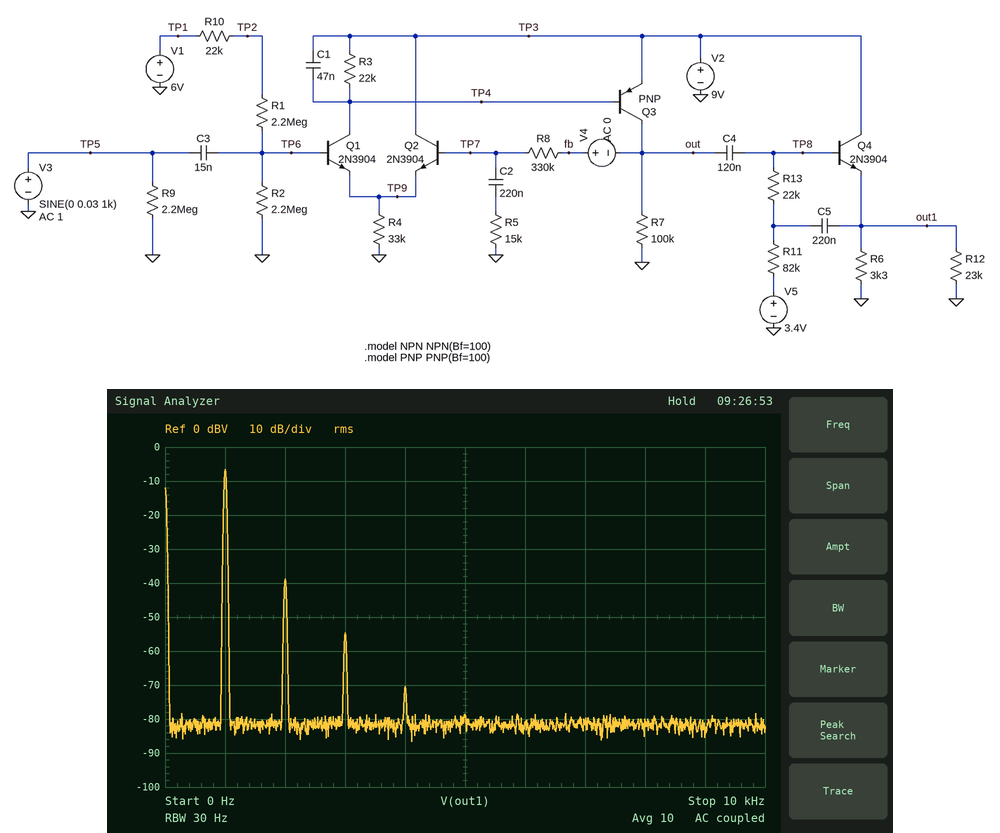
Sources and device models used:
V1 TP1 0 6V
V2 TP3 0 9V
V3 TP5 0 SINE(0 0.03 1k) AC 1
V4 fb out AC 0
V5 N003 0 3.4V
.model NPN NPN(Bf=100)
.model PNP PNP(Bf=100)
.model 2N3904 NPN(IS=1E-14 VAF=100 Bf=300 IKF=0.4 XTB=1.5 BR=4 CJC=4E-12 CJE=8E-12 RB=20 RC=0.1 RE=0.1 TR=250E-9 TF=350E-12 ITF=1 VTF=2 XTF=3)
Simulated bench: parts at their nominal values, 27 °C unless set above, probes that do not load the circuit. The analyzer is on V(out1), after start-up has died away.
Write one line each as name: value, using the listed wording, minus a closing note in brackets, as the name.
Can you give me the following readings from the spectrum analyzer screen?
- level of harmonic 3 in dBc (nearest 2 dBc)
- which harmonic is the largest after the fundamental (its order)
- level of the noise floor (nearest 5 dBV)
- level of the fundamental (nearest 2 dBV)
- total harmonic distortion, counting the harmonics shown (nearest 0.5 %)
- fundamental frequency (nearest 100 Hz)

level of harmonic 3 in dBc: -48 dBc
which harmonic is the largest after the fundamental: 2
level of the noise floor: -80 dBV
level of the fundamental: -6 dBV
total harmonic distortion, counting the harmonics shown: 2.5 %
fundamental frequency: 1.0 kHz
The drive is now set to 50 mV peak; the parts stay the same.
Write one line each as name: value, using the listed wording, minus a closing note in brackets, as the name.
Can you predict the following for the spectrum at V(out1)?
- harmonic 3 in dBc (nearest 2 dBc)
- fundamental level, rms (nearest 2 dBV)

harmonic 3 in dBc: -38 dBc
fundamental level, rms: -2 dBV
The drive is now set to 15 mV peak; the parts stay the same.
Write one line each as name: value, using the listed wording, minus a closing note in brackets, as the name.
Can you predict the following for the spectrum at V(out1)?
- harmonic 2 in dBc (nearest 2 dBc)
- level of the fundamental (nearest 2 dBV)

harmonic 2 in dBc: -38 dBc
level of the fundamental: -12 dBV
